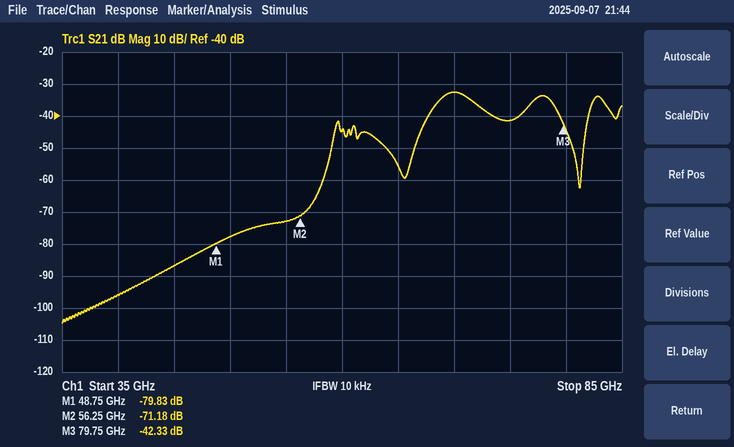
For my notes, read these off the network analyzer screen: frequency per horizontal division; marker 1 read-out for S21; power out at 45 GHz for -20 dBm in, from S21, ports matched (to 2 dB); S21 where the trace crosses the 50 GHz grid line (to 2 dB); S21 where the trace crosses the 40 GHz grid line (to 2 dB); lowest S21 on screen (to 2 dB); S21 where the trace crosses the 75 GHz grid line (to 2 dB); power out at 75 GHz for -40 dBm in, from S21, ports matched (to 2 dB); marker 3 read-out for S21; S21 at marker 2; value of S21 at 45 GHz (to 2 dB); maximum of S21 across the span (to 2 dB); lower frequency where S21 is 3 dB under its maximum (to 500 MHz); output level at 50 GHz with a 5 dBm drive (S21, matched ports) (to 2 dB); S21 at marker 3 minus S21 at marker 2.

5 GHz
-79.83 dB
-106 dBm
-78 dB
-96 dB
-104 dB
-42 dB
-82 dBm
-42.33 dB
-71.18 dB
-86 dB
-32 dB
68.5 GHz
-72 dBm
28.85 dB
